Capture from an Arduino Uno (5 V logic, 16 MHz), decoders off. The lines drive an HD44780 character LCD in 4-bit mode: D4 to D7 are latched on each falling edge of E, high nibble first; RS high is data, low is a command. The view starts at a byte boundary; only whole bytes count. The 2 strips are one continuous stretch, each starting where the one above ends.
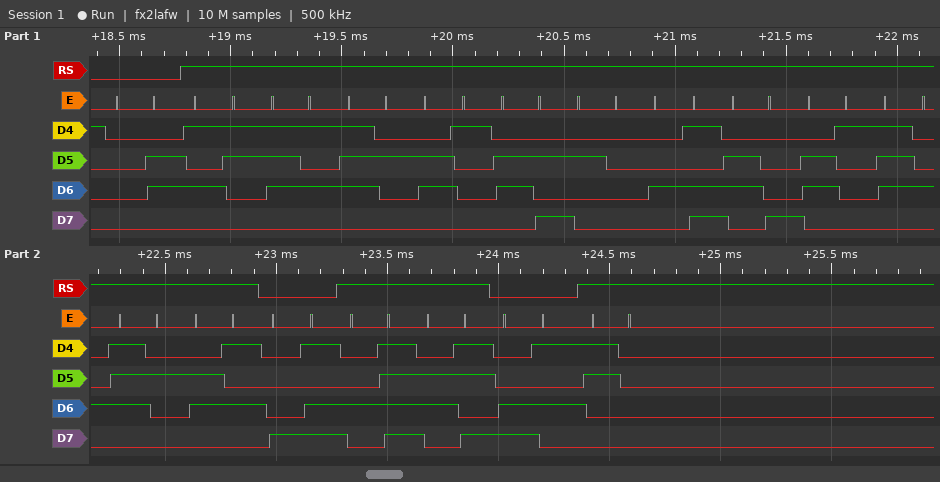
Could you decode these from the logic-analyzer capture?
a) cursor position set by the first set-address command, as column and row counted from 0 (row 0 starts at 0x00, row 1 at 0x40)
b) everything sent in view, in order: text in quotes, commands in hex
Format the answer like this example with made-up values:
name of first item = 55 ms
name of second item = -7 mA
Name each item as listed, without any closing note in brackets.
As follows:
cursor position set by the first set-address command, as column and row counted from 0 = column 13, row 0
everything sent in view, in order: text in quotes, commands in hex = 0x06 "Suraj Mhatre" 0x8D "Ok" 0xC5 "0"
